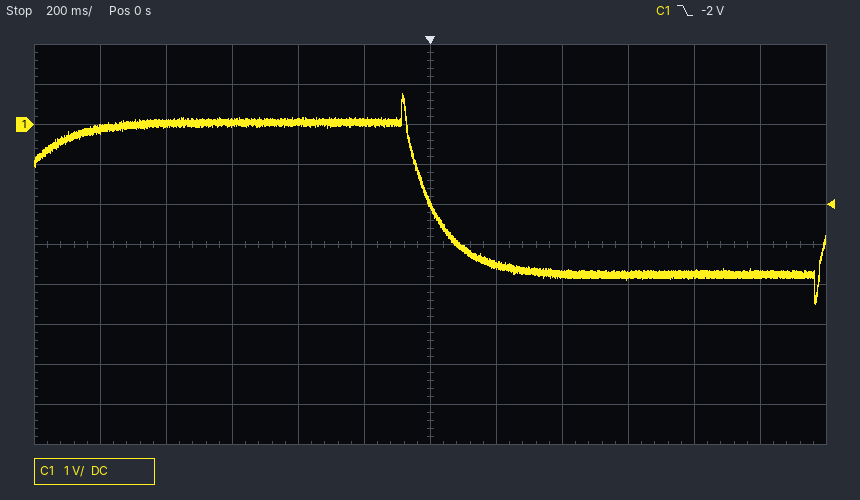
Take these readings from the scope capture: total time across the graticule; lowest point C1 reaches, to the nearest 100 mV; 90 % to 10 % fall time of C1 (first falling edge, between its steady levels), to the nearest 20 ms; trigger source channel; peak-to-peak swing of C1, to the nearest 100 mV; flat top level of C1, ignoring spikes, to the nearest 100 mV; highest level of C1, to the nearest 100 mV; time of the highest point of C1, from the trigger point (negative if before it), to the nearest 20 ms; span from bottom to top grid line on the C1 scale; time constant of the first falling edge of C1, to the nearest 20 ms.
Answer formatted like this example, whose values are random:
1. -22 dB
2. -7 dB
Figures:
1. 2.4 s
2. -4.5 V
3. 220 ms
4. C1
5. 5.3 V
6. 0.0 V
7. 800 mV
8. -80 ms
9. 10 V
10. 100 ms
